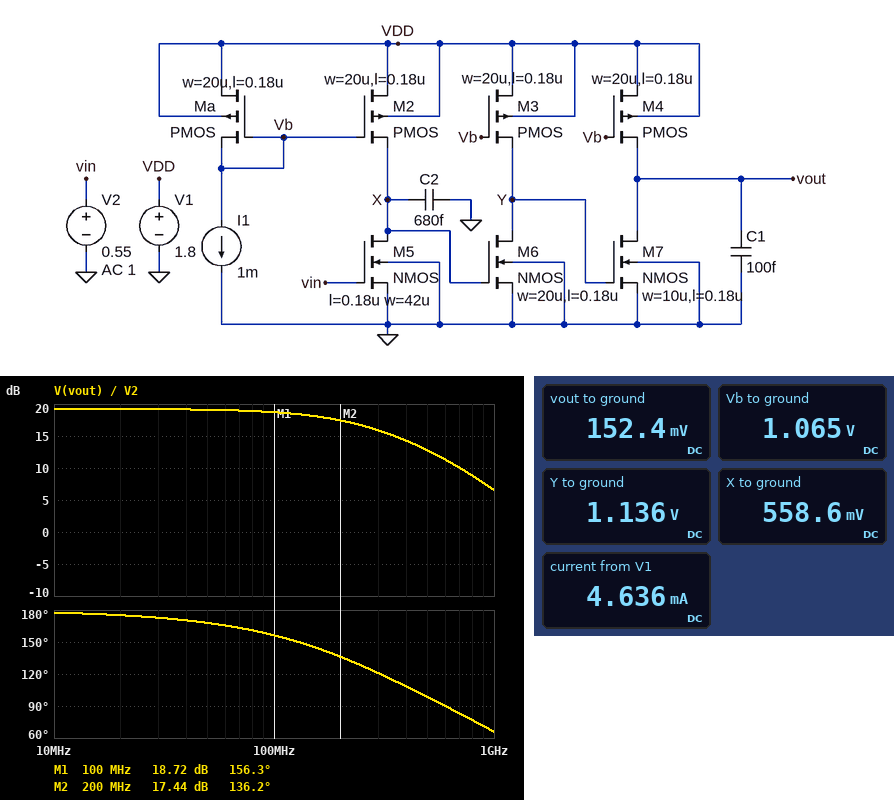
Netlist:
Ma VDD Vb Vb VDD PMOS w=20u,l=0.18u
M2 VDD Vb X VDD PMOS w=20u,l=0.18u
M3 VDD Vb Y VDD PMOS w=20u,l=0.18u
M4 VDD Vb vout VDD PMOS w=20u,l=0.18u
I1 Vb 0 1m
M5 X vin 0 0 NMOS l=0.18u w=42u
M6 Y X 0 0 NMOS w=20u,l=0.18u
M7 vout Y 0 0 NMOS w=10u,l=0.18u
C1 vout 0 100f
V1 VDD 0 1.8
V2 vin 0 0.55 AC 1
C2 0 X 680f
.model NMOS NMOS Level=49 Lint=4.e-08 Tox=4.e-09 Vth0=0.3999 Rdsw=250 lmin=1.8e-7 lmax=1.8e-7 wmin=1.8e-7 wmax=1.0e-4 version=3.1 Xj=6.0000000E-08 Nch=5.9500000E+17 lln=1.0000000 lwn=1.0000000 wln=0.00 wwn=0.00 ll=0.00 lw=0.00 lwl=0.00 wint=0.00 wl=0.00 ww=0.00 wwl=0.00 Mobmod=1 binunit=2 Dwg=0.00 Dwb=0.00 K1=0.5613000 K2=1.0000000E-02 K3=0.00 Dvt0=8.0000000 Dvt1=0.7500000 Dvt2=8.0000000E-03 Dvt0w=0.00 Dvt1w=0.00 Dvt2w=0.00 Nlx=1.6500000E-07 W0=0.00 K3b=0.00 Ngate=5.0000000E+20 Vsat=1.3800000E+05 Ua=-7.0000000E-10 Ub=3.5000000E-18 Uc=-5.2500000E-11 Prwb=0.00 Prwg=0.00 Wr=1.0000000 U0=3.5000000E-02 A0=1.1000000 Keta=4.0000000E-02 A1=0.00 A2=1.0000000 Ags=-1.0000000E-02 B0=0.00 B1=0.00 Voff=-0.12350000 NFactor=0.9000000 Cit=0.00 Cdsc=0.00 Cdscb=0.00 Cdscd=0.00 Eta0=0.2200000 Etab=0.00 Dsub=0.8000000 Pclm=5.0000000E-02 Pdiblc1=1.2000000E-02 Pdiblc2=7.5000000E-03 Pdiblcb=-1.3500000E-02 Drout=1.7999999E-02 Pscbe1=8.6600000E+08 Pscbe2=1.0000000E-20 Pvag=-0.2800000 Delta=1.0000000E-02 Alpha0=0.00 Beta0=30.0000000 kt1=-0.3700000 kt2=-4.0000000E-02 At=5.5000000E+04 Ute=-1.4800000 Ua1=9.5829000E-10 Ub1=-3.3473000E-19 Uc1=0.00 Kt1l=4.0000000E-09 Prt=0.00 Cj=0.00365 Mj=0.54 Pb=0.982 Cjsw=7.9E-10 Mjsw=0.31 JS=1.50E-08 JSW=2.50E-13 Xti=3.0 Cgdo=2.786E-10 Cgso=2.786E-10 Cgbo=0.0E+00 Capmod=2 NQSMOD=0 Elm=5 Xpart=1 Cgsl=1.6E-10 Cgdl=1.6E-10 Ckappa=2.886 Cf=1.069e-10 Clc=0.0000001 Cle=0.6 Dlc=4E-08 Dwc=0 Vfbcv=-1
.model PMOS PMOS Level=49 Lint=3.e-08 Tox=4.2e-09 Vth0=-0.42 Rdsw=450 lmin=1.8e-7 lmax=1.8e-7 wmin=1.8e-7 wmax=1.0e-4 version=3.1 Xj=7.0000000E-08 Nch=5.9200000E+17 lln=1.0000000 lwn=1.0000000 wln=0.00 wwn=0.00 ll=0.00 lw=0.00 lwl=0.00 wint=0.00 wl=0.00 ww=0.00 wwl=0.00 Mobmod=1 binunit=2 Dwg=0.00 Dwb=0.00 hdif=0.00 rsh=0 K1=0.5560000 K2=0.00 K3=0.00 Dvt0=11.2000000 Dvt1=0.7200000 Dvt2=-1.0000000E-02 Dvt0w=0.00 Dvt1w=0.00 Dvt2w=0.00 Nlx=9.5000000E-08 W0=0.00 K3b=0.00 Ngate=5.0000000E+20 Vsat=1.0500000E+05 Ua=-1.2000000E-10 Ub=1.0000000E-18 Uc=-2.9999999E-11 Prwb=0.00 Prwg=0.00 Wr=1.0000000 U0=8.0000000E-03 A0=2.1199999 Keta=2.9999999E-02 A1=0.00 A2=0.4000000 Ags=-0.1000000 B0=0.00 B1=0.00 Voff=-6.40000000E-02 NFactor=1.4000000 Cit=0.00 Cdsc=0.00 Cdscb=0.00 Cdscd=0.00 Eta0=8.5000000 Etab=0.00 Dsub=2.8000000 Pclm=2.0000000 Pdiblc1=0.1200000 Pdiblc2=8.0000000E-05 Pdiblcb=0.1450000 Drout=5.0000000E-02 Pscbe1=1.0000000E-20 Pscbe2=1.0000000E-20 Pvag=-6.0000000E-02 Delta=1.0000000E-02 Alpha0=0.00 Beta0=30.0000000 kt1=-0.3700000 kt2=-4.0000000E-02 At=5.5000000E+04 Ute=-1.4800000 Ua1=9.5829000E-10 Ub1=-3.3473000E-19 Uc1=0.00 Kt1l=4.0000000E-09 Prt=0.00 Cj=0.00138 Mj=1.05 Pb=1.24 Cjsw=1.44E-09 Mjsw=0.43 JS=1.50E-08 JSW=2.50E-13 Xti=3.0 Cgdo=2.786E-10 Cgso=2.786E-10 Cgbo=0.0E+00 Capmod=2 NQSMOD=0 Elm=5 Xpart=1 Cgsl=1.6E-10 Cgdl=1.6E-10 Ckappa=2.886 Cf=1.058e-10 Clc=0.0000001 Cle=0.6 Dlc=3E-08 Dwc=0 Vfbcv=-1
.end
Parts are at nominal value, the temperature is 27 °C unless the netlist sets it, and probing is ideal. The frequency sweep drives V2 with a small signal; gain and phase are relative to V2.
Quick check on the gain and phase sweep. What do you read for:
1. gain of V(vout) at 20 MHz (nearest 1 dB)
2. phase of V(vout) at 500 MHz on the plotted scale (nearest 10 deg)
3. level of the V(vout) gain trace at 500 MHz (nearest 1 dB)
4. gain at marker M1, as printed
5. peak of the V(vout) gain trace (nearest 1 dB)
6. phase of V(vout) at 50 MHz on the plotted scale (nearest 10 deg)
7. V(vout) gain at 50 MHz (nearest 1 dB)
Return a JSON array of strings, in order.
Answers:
["19 dB", "100 deg", "13 dB", "18.72 dB", "19 dB", "170 deg", "19 dB"]
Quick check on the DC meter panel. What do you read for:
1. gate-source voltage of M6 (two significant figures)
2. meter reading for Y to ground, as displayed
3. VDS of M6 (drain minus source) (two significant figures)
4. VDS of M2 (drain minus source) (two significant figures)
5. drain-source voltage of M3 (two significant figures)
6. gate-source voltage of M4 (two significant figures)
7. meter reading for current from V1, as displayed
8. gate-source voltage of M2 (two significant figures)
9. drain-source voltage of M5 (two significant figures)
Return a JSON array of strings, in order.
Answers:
["560 mV", "1.136 V", "1.1 V", "1.2 V", "660 mV", "910 mV", "4.636 mA", "510 mV", "560 mV"]
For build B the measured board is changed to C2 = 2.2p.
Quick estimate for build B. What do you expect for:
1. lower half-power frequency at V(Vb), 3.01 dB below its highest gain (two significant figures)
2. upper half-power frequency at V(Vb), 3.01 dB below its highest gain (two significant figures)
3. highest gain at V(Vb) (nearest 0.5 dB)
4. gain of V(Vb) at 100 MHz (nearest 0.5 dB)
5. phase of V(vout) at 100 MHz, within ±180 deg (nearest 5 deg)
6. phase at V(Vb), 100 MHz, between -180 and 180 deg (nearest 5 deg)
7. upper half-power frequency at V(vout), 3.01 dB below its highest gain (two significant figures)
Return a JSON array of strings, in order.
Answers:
["89 MHz", "1.5 GHz", "-24.5 dB", "-27.0 dB", "130 deg", "40 deg", "100 MHz"]
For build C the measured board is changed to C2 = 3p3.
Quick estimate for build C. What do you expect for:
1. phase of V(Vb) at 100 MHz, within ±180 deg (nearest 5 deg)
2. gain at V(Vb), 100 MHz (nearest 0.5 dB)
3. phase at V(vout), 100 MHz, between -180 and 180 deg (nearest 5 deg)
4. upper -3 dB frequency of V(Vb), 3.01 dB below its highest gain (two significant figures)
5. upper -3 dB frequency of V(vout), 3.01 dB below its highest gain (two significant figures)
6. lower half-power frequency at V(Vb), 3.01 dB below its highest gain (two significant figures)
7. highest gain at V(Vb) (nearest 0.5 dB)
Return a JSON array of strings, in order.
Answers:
["30 deg", "-29.0 dB", "120 deg", "1.5 GHz", "68 MHz", "63 MHz", "-27.5 dB"]
